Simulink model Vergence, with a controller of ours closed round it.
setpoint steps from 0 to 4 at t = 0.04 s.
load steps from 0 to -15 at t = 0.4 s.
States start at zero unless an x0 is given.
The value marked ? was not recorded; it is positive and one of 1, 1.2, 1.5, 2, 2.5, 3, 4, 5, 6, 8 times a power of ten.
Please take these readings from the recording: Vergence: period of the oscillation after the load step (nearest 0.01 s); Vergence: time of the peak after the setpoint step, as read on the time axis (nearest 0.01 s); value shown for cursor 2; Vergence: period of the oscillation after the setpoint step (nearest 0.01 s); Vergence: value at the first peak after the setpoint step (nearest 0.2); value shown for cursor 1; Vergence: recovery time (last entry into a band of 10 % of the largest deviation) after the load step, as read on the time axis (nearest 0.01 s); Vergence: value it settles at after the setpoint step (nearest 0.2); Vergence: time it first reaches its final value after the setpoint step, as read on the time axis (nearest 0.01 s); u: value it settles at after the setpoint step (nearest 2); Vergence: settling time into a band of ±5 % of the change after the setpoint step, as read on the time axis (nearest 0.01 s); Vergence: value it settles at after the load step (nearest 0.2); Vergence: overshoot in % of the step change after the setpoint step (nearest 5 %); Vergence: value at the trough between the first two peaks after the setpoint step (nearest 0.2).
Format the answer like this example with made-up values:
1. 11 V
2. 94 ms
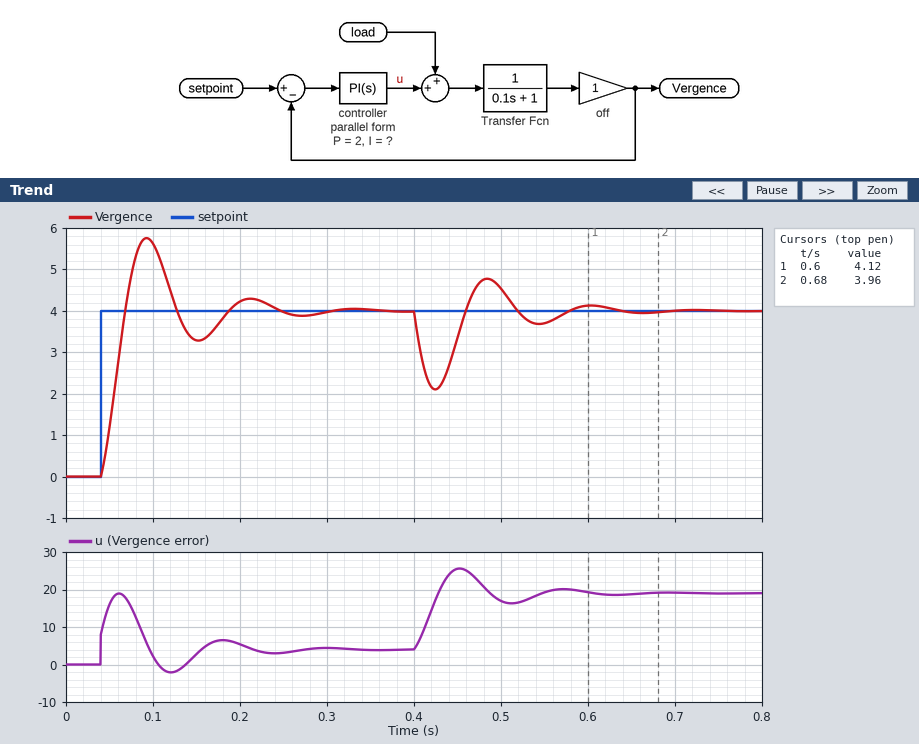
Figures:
1. 0.12 s
2. 0.09 s
3. 3.96
4. 0.12 s
5. 5.8
6. 4.12
7. 0.56 s
8. 4.0
9. 0.07 s
10. 4
11. 0.23 s
12. 4.0
13. 45 %
14. 3.2
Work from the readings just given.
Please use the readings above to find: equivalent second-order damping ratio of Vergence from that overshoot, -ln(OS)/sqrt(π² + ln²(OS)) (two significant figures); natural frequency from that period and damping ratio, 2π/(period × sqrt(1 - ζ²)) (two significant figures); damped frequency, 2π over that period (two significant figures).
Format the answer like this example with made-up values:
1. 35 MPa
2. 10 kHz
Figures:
1. 0.25
2. 54 rad/s
3. 52 rad/s
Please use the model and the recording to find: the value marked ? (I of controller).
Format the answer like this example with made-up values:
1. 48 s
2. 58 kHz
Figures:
1. 300
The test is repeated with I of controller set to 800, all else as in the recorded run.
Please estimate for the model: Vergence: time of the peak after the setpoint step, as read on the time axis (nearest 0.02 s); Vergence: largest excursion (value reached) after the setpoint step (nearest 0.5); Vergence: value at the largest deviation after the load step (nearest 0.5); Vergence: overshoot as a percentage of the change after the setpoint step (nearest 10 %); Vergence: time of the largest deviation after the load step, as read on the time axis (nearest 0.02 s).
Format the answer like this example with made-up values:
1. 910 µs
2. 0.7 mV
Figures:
1. 0.08 s
2. 6.5
3. 2.5
4. 60 %
5. 0.42 s
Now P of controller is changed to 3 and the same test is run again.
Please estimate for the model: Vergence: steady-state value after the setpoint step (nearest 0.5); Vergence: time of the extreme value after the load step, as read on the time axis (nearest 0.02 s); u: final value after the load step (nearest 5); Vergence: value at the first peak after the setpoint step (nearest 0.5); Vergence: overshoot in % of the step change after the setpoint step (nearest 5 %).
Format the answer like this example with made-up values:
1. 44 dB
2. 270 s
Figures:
1. 4.0
2. 0.42 s
3. 20
4. 5.5
5. 35 %
